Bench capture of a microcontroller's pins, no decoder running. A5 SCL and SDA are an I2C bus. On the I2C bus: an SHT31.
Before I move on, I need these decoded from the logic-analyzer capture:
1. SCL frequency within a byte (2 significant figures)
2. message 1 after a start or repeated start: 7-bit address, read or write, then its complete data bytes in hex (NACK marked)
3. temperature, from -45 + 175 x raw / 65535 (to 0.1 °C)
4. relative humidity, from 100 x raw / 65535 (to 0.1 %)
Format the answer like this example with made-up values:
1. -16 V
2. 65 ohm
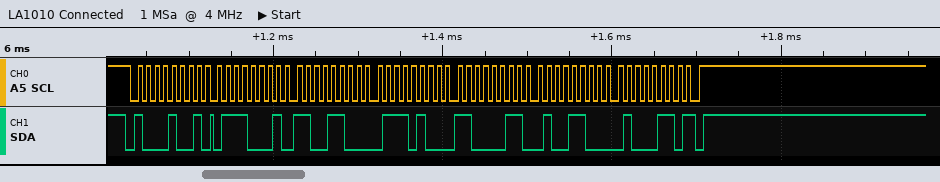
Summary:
1. 100 kHz
2. 0x44 read: 71 CC 74 C3 4C 46 NACK
3. 32.8 °C
4. 76.3 %
